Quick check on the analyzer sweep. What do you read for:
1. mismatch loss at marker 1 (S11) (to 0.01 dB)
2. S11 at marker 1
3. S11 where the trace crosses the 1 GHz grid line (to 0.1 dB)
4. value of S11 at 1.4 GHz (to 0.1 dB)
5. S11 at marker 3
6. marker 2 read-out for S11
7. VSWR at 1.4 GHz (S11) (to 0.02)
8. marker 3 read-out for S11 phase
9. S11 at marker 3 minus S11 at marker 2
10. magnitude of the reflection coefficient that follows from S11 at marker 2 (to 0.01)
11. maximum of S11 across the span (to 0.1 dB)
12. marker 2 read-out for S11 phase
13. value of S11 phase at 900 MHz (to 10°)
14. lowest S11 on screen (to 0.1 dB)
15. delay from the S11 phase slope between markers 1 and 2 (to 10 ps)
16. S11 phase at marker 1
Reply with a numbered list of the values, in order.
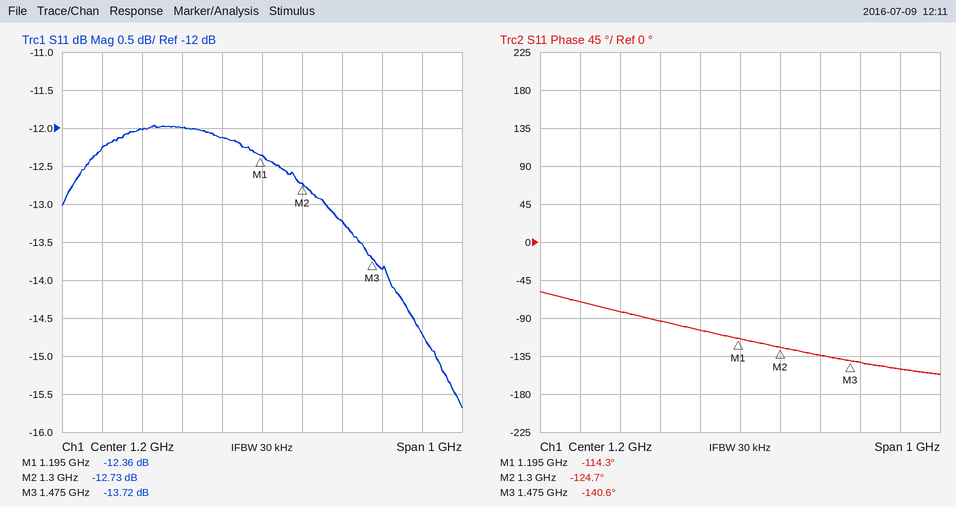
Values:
1. 0.26 dB
2. -12.36 dB
3. -12.0 dB
4. -13.2 dB
5. -13.72 dB
6. -12.73 dB
7. 1.56
8. -140.6°
9. -0.99 dB
10. 0.23
11. -12.0 dB
12. -124.7°
13. -80°
14. -15.7 dB
15. 280 ps
16. -114.3°
